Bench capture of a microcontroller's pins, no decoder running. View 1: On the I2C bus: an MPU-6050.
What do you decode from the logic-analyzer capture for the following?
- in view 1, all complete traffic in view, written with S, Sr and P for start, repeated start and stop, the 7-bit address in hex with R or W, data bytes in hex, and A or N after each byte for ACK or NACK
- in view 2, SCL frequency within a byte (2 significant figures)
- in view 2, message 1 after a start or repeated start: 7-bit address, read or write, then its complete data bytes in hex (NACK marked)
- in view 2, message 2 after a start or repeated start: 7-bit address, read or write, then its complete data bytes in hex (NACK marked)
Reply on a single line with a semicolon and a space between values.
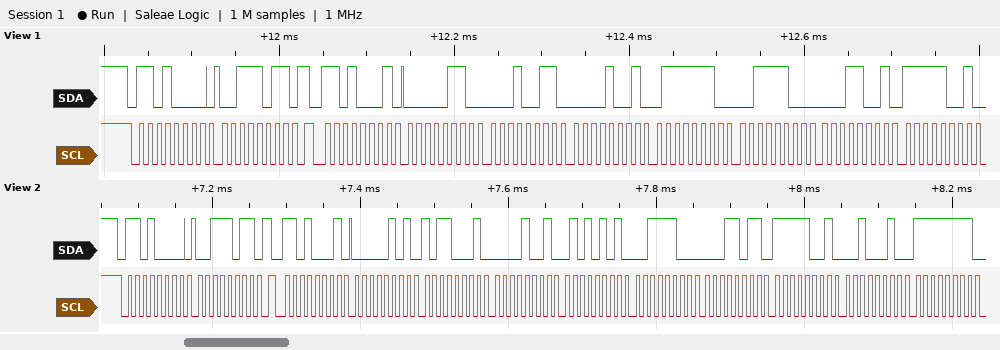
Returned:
S 68W A 3B A Sr 68R A 06 A 13 A 09 A 7E A 3C A 19 A F9 A; 100 kHz; 0x68 write: 3B; 0x68 read: 05 B1 09 55 3C 1B F9 22 FF
